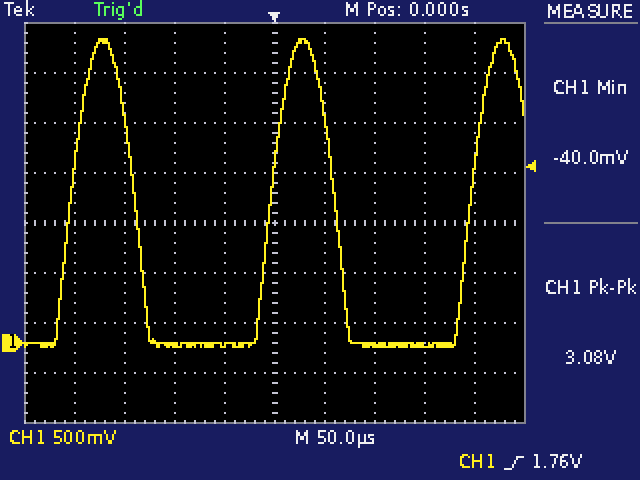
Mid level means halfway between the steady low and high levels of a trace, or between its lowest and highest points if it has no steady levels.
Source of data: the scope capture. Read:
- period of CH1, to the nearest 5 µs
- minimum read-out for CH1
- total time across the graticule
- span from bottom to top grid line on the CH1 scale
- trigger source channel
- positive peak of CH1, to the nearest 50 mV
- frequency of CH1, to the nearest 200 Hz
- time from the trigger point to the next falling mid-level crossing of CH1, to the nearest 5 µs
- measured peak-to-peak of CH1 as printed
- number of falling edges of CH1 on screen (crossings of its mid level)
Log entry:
200 µs
-40.0 mV
500 µs
4 V
CH1
3.05 V
5.0 kHz
60 µs
3.08 V
2
